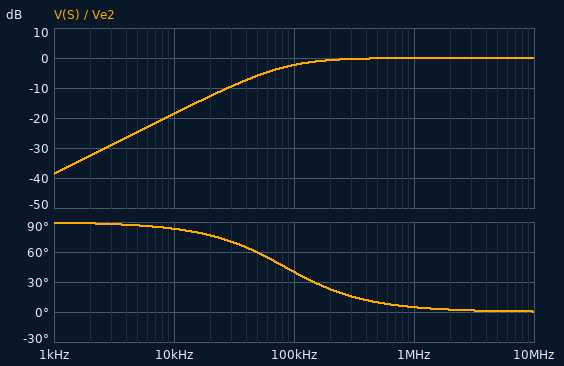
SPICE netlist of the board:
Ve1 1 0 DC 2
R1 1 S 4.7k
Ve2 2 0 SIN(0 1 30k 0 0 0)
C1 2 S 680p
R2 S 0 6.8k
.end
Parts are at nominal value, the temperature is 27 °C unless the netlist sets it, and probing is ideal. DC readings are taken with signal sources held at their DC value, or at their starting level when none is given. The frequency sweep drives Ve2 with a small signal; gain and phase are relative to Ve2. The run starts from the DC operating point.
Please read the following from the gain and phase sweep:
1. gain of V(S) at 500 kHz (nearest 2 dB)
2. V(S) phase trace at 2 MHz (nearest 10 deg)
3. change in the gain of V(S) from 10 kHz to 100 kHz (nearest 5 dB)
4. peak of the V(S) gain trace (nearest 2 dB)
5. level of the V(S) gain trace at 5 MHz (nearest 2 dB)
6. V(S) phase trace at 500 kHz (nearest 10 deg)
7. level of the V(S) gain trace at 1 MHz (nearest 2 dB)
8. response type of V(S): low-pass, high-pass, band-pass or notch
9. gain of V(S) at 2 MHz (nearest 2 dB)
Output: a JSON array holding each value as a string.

["0 dB", "0 deg", "15 dB", "0 dB", "0 dB", "10 deg", "0 dB", "high-pass", "0 dB"]
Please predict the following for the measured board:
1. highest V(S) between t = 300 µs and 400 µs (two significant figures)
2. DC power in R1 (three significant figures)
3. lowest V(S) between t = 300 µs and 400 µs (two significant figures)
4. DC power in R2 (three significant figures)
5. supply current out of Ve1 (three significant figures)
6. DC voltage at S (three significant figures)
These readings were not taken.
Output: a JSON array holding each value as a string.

["1.5 V", "142 µW", "850 mV", "206 µW", "174 µA", "1.18 V"]
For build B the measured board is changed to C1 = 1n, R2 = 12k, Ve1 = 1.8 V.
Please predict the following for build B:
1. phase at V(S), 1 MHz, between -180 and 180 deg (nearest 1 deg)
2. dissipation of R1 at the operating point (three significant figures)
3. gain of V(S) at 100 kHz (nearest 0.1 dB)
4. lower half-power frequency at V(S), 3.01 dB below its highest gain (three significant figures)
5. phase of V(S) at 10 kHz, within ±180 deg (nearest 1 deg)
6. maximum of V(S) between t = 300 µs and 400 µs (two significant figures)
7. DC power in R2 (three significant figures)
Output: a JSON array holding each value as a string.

["3 deg", "54.6 µW", "-0.9 dB", "47.1 kHz", "78 deg", "1.8 V", "139 µW"]
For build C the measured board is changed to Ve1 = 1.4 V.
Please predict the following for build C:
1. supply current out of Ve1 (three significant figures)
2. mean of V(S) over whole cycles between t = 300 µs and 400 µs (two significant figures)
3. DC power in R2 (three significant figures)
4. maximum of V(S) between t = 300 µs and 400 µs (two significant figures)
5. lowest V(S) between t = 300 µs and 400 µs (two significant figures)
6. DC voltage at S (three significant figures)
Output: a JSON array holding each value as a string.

["122 µA", "830 mV", "101 µW", "1.2 V", "490 mV", "828 mV"]
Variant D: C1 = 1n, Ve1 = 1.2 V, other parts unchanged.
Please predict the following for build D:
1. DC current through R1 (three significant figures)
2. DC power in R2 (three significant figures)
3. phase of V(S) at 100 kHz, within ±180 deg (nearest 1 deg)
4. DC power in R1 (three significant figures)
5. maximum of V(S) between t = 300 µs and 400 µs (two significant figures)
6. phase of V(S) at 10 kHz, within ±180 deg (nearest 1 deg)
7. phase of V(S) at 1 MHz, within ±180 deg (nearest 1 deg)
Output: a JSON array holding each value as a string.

["104 µA", "74.0 µW", "30 deg", "51.2 µW", "1.2 V", "80 deg", "3 deg"]
